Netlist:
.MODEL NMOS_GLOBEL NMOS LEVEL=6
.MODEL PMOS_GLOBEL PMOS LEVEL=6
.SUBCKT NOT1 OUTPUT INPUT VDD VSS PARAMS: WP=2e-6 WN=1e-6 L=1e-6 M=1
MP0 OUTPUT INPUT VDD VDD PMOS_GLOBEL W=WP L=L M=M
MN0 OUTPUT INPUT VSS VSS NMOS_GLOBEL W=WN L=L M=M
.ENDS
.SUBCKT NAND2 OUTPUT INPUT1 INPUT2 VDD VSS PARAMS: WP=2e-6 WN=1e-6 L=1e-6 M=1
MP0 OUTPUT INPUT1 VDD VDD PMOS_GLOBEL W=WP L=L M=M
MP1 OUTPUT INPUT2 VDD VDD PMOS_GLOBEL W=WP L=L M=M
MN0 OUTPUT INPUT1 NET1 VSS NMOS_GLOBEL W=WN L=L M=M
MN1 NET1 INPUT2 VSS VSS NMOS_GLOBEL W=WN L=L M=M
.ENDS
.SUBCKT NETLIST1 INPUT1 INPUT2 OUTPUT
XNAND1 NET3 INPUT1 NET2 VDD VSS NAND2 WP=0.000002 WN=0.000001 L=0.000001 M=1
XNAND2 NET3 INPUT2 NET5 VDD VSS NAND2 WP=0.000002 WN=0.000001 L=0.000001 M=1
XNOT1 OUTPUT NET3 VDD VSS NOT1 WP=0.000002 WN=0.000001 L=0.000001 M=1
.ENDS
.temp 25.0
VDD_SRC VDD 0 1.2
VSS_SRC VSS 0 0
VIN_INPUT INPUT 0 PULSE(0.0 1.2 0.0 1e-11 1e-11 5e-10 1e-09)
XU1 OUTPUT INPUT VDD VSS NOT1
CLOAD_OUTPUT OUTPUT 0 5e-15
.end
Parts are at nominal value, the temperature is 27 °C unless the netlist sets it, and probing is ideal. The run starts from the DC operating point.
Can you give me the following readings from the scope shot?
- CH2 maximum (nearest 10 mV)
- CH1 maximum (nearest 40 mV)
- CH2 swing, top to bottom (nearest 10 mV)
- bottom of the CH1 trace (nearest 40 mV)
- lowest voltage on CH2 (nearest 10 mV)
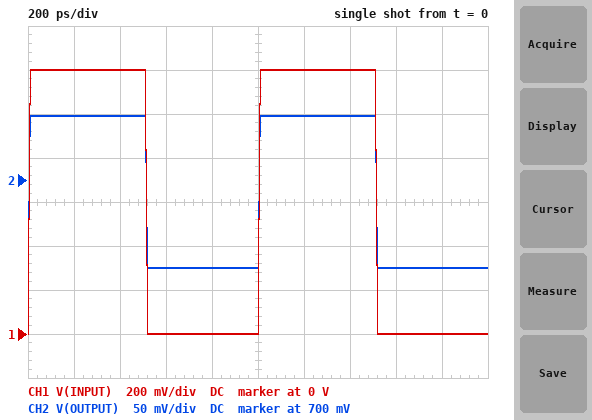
770 mV
1.20 V
170 mV
0 V
600 mV
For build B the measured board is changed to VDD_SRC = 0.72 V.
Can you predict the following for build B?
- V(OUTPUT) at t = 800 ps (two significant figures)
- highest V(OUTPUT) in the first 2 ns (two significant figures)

360 mV
530 mV
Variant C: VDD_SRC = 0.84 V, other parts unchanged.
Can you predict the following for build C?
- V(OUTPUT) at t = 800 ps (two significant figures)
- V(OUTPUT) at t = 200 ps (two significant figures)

420 mV
590 mV
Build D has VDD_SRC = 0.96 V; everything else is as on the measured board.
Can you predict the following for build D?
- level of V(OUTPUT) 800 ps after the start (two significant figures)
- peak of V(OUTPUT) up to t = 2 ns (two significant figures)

480 mV
650 mV
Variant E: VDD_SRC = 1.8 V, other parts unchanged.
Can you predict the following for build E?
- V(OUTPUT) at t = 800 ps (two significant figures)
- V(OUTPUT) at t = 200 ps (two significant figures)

1.8 V
2.0 V
